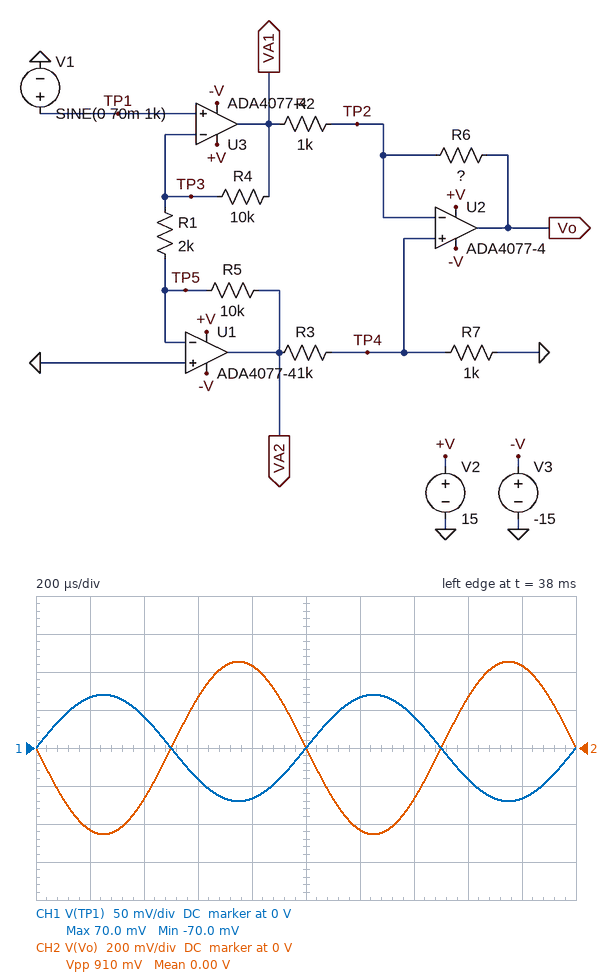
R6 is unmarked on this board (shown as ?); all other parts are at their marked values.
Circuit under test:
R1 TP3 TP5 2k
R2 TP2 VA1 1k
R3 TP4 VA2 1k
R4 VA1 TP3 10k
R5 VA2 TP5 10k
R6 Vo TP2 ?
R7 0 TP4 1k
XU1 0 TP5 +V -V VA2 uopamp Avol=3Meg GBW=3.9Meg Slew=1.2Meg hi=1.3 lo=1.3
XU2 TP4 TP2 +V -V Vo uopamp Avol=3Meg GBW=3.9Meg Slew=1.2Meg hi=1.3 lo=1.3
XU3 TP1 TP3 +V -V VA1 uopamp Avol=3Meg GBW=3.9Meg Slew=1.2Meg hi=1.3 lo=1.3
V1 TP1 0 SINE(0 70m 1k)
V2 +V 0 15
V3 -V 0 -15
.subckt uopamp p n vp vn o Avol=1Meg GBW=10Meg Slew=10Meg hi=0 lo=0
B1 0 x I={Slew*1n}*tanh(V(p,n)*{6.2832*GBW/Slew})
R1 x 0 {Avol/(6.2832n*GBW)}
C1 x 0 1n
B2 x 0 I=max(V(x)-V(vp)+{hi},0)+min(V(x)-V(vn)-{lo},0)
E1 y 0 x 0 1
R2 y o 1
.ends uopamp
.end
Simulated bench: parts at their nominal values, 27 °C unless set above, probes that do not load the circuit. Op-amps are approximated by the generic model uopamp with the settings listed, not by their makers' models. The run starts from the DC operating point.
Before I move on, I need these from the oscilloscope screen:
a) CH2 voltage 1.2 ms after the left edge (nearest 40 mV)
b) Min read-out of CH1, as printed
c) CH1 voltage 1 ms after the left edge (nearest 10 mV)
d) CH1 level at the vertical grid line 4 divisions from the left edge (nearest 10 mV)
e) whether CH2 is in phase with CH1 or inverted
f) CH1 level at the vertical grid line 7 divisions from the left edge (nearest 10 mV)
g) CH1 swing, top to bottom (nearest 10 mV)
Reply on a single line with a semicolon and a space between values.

-440 mV; -70.0 mV; 0 V; -70 mV; inverted; 40 mV; 140 mV
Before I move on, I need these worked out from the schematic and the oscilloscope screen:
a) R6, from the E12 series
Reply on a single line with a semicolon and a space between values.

470 Ω
